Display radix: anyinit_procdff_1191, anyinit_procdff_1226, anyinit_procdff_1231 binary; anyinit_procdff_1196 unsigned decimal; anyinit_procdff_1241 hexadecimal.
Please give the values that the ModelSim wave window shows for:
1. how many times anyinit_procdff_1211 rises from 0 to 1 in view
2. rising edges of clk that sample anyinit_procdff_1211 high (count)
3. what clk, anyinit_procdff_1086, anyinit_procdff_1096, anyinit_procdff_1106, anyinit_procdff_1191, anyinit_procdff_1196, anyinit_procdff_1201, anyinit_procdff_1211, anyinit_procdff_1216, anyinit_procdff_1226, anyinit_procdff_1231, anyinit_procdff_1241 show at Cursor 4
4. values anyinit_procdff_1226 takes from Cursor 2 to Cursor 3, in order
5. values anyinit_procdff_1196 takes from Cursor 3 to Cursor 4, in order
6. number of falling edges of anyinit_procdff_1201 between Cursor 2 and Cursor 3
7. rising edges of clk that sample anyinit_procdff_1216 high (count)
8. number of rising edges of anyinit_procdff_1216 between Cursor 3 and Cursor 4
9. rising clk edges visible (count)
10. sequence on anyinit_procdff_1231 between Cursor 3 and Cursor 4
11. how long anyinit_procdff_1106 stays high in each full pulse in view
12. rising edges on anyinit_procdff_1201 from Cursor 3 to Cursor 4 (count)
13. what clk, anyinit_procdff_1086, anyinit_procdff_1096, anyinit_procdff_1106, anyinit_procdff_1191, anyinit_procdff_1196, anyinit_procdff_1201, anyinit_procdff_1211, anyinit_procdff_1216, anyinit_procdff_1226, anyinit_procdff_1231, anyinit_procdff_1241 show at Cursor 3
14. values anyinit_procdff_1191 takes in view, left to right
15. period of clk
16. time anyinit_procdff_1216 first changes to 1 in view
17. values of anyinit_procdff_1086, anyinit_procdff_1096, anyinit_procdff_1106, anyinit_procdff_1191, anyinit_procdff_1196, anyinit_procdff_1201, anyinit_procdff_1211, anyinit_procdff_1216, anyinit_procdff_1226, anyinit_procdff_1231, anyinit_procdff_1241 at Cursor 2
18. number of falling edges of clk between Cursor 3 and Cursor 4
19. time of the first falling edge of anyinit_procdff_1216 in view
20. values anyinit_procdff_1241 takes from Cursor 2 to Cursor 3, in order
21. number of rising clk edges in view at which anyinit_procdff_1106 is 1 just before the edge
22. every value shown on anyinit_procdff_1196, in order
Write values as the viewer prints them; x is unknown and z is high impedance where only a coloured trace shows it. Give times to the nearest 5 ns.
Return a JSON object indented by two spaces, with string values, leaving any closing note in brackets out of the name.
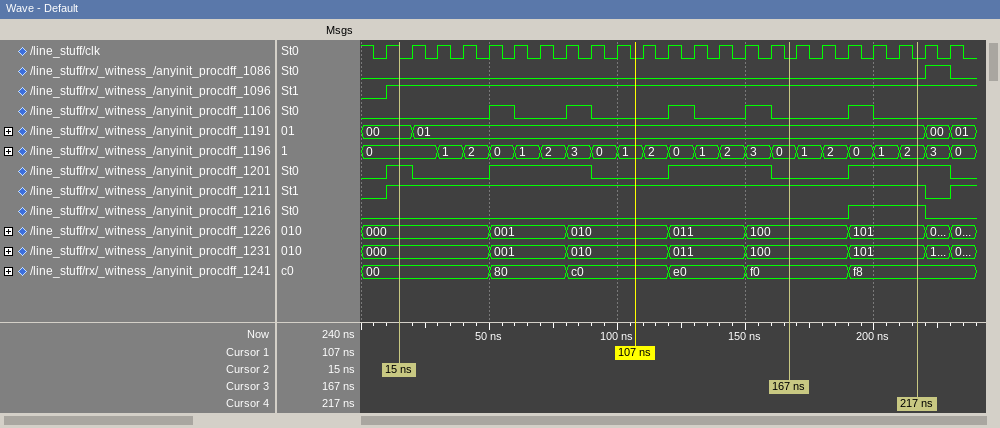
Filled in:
{
  "how many times anyinit_procdff_1211 rises from 0 to 1 in view": "2",
  "rising edges of clk that sample anyinit_procdff_1211 high": "21",
  "what clk, anyinit_procdff_1086, anyinit_procdff_1096, anyinit_procdff_1106, anyinit_procdff_1191, anyinit_procdff_1196, anyinit_procdff_1201, anyinit_procdff_1211, anyinit_procdff_1216, anyinit_procdff_1226, anyinit_procdff_1231, anyinit_procdff_1241 show at Cursor 4": "clk=0, anyinit_procdff_1086=0, anyinit_procdff_1096=1, anyinit_procdff_1106=0, anyinit_procdff_1191=01, anyinit_procdff_1196=2, anyinit_procdff_1201=1, anyinit_procdff_1211=1, anyinit_procdff_1216=1, anyinit_procdff_1226=101, anyinit_procdff_1231=101, anyinit_procdff_1241=f8",
  "values anyinit_procdff_1226 takes from Cursor 2 to Cursor 3, in order": "000, 001, 010, 011, 100",
  "values anyinit_procdff_1196 takes from Cursor 3 to Cursor 4, in order": "0, 1, 2, 0, 1, 2",
  "number of falling edges of anyinit_procdff_1201 between Cursor 2 and Cursor 3": "3",
  "rising edges of clk that sample anyinit_procdff_1216 high": "3",
  "number of rising edges of anyinit_procdff_1216 between Cursor 3 and Cursor 4": "1",
  "rising clk edges visible": "23",
  "sequence on anyinit_procdff_1231 between Cursor 3 and Cursor 4": "100, 101",
  "how long anyinit_procdff_1106 stays high in each full pulse in view": "10 ns, 10 ns, 10 ns, 10 ns, 10 ns",
  "rising edges on anyinit_procdff_1201 from Cursor 3 to Cursor 4": "1",
  "what clk, anyinit_procdff_1086, anyinit_procdff_1096, anyinit_procdff_1106, anyinit_procdff_1191, anyinit_procdff_1196, anyinit_procdff_1201, anyinit_procdff_1211, anyinit_procdff_1216, anyinit_procdff_1226, anyinit_procdff_1231, anyinit_procdff_1241 show at Cursor 3": "clk=0, anyinit_procdff_1086=0, anyinit_procdff_1096=1, anyinit_procdff_1106=0, anyinit_procdff_1191=01, anyinit_procdff_1196=0, anyinit_procdff_1201=0, anyinit_procdff_1211=1, anyinit_procdff_1216=0, anyinit_procdff_1226=100, anyinit_procdff_1231=100, anyinit_procdff_1241=f0",
  "values anyinit_procdff_1191 takes in view, left to right": "00, 01, 00, 01",
  "period of clk": "10 ns",
  "time anyinit_procdff_1216 first changes to 1 in view": "190 ns",
  "values of anyinit_procdff_1086, anyinit_procdff_1096, anyinit_procdff_1106, anyinit_procdff_1191, anyinit_procdff_1196, anyinit_procdff_1201, anyinit_procdff_1211, anyinit_procdff_1216, anyinit_procdff_1226, anyinit_procdff_1231, anyinit_procdff_1241 at Cursor 2": "anyinit_procdff_1086=0, anyinit_procdff_1096=1, anyinit_procdff_1106=0, anyinit_procdff_1191=00, anyinit_procdff_1196=0, anyinit_procdff_1201=1, anyinit_procdff_1211=1, anyinit_procdff_1216=0, anyinit_procdff_1226=000, anyinit_procdff_1231=000, anyinit_procdff_1241=00",
  "number of falling edges of clk between Cursor 3 and Cursor 4": "5",
  "time of the first falling edge of anyinit_procdff_1216 in view": "220 ns",
  "values anyinit_procdff_1241 takes from Cursor 2 to Cursor 3, in order": "00, 80, c0, e0, f0",
  "number of rising clk edges in view at which anyinit_procdff_1106 is 1 just before the edge": "5",
  "every value shown on anyinit_procdff_1196, in order": "0, 1, 2, 0, 1, 2, 3, 0, 1, 2, 0, 1, 2, 3, 0, 1, 2, 0, 1, 2, 3, 0"
}
